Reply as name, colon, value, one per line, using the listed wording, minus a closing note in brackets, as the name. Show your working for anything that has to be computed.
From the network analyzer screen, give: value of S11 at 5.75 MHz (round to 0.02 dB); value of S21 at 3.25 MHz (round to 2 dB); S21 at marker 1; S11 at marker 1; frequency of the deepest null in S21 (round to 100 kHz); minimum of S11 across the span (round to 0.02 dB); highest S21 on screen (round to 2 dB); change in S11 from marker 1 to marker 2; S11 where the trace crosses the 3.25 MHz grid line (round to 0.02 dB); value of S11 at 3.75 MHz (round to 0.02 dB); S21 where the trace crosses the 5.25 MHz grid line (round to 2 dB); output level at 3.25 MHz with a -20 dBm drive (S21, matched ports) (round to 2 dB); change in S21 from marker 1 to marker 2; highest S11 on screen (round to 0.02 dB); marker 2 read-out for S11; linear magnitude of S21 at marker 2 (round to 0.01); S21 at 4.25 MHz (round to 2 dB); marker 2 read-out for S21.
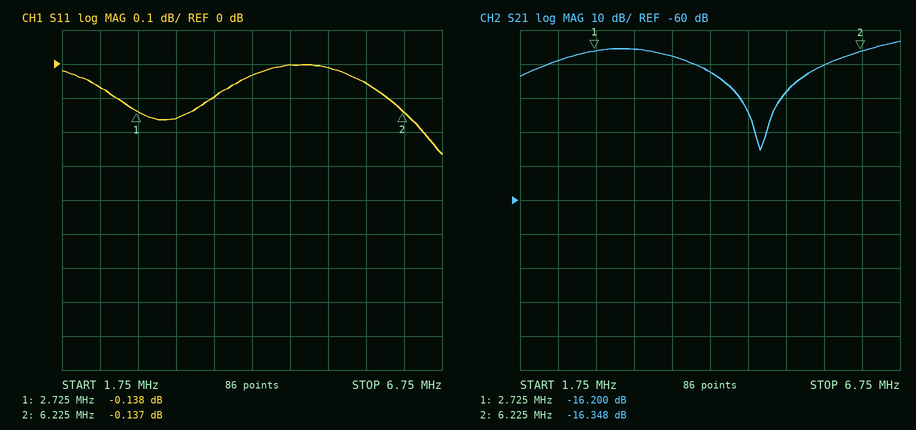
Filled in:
value of S11 at 5.75 MHz: -0.06 dB
value of S21 at 3.25 MHz: -16 dB
S21 at marker 1: -16.200 dB
S11 at marker 1: -0.138 dB
frequency of the deepest null in S21: 4.9 MHz
minimum of S11 across the span: -0.26 dB
highest S21 on screen: -14 dB
change in S11 from marker 1 to marker 2: -0.137 − (-0.138) = 0.001 dB
S11 where the trace crosses the 3.25 MHz grid line: -0.16 dB
value of S11 at 3.75 MHz: -0.10 dB
S21 where the trace crosses the 5.25 MHz grid line: -28 dB
output level at 3.25 MHz with a -20 dBm drive (S21, matched ports): -20 dBm + (-16 dB) = -36 dBm
change in S21 from marker 1 to marker 2: -16.348 − (-16.2) = -0.148 dB
highest S11 on screen: 0.00 dB
marker 2 read-out for S11: -0.137 dB
linear magnitude of S21 at marker 2: 10^(-16.348/20) ≈ 0.15
S21 at 4.25 MHz: -22 dB
marker 2 read-out for S21: -16.348 dB
